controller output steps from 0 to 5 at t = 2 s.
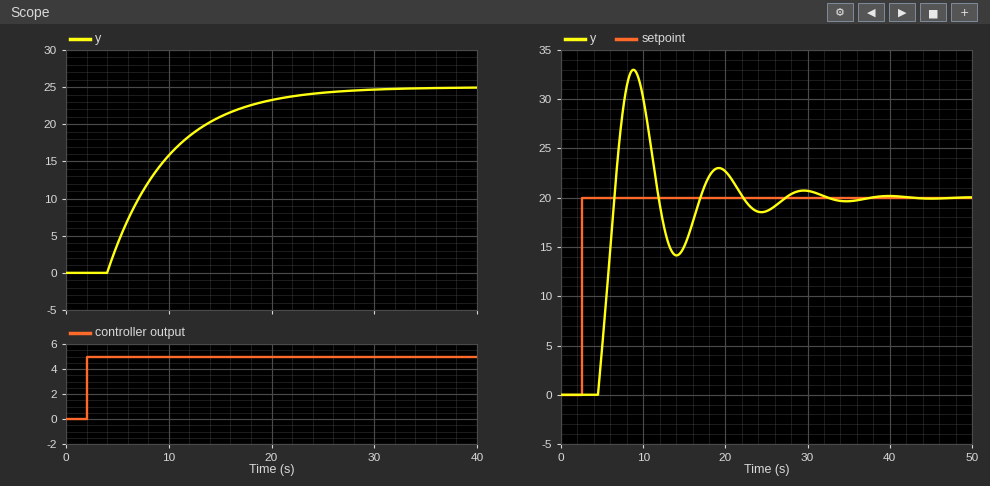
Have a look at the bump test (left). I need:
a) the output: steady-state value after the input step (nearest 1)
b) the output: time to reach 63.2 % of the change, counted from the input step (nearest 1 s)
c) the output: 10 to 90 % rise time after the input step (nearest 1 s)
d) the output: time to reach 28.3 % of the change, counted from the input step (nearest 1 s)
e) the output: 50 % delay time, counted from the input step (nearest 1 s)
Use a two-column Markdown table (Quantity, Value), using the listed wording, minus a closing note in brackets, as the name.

| Quantity | Value |
|---|---|
| the output: steady-state value after the input step | 25 |
| the output: time to reach 63.2 % of the change, counted from the input step | 8 s |
| the output: 10 to 90 % rise time after the input step | 13 s |
| the output: time to reach 28.3 % of the change, counted from the input step | 4 s |
| the output: 50 % delay time, counted from the input step | 6 s |
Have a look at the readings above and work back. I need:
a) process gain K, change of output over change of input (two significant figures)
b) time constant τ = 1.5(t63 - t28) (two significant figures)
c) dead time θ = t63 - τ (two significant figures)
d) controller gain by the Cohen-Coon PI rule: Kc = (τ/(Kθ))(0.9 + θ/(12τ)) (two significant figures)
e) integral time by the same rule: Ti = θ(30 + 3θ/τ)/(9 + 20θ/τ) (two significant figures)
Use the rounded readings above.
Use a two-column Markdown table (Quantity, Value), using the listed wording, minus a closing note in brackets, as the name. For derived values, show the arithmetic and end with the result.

| Quantity | Value |
|---|---|
| process gain K, change of output over change of input | (25 - 0) / 5 = 5.0 |
| time constant τ = 1.5(t63 - t28) | 1.5 × (8 - 4) = 6.0 s |
| dead time θ = t63 - τ | 8 - 6 = 2.0 s |
| controller gain by the Cohen-Coon PI rule: Kc = (τ/(Kθ))(0.9 + θ/(12τ)) | 6 / (5 × 2) × (0.9 + 2 / (12 × 6)) = 0.56 |
| integral time by the same rule: Ti = θ(30 + 3θ/τ)/(9 + 20θ/τ) | 2 × (30 + 3 × 2 / 6) / (9 + 20 × 2 / 6) = 4.0 s |
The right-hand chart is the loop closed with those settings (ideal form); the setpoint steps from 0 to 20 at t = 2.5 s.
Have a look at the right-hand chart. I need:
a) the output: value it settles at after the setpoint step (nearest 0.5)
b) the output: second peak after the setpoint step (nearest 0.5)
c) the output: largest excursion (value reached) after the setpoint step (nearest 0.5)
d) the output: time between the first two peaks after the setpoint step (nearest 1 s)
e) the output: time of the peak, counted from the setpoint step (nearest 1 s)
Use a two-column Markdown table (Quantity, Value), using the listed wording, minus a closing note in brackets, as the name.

| Quantity | Value |
|---|---|
| the output: value it settles at after the setpoint step | 20.0 |
| the output: second peak after the setpoint step | 23.0 |
| the output: largest excursion (value reached) after the setpoint step | 33.0 |
| the output: time between the first two peaks after the setpoint step | 10 s |
| the output: time of the peak, counted from the setpoint step | 6 s |
